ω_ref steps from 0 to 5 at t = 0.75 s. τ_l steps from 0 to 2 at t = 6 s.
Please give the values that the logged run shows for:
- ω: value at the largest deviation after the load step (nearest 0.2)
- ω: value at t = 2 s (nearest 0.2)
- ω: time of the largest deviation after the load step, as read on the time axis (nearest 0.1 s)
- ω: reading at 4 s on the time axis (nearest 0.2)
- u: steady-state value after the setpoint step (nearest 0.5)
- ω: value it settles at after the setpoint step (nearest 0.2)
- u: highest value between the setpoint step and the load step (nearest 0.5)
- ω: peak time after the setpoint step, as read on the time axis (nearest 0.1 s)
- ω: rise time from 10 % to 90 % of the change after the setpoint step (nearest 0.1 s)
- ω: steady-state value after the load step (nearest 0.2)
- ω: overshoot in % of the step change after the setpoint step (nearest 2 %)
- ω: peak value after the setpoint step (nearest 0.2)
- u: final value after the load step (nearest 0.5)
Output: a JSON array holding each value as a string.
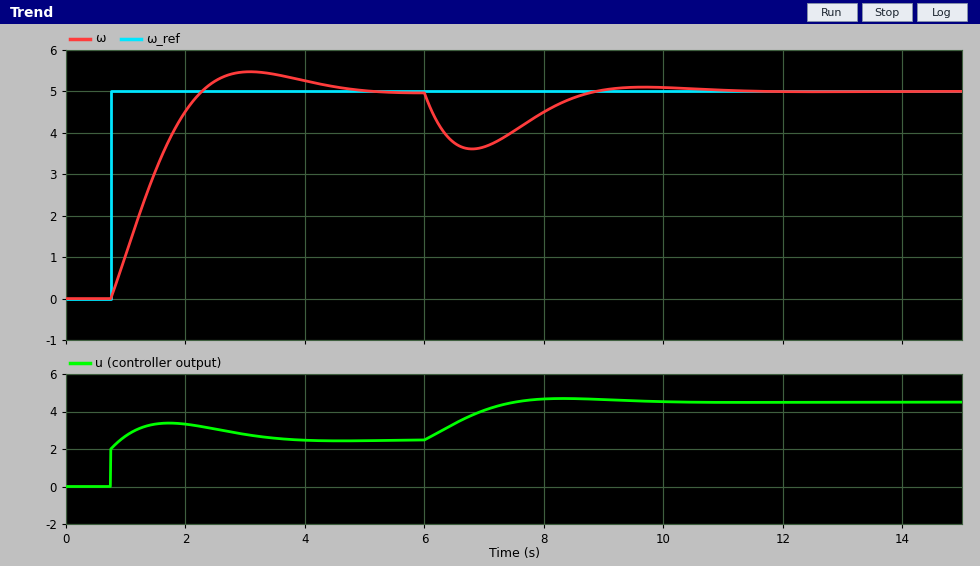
["3.6", "4.6", "6.8 s", "5.2", "2.5", "5.0", "3.5", "3.1 s", "1.1 s", "5.0", "10 %", "5.4", "4.5"]
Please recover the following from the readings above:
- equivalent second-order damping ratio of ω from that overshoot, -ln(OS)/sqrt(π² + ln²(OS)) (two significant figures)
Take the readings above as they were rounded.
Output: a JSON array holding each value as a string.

["0.59"]
